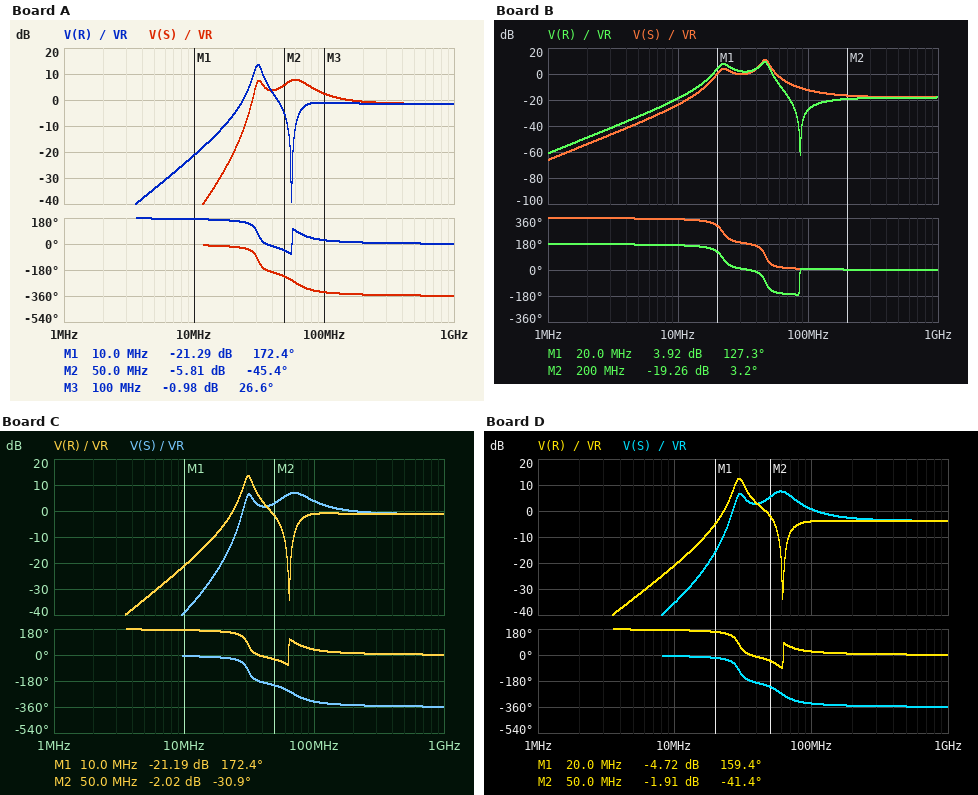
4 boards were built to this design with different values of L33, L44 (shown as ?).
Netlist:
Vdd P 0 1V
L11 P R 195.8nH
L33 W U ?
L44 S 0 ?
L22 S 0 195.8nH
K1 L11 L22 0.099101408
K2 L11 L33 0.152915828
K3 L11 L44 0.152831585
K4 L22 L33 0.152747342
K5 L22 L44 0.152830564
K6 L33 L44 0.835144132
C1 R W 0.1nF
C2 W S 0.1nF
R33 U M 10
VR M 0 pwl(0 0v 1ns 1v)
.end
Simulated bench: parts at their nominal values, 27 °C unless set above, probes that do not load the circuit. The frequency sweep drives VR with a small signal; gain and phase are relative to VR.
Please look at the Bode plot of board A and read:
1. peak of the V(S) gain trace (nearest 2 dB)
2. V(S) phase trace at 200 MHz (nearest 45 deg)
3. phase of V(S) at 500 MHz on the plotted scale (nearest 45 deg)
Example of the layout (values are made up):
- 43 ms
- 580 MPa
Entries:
- 8 dB
- -360 deg
- -360 deg
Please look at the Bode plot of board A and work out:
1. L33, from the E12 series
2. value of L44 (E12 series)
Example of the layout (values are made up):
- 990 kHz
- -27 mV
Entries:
- 82 nH
- 330 nH
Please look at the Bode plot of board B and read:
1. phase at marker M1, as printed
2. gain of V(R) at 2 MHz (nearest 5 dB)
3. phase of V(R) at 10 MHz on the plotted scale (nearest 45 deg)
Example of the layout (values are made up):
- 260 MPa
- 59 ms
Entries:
- 127.3 deg
- -50 dB
- 180 deg
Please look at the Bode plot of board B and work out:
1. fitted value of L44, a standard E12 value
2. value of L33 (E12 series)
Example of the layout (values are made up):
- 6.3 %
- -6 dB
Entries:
- 560 nH
- 470 nH
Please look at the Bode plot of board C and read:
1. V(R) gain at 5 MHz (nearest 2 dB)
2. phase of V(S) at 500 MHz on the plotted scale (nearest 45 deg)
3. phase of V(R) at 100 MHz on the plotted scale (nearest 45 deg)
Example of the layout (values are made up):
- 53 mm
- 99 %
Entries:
- -34 dB
- -360 deg
- 45 deg
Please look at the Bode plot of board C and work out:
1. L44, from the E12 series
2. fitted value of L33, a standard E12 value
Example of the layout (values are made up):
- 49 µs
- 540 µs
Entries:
- 220 nH
- 68 nH
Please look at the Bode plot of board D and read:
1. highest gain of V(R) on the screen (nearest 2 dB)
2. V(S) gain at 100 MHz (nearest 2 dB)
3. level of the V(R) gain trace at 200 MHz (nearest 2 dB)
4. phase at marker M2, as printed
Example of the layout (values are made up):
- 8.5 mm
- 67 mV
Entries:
- 12 dB
- 0 dB
- -4 dB
- -41.4 deg
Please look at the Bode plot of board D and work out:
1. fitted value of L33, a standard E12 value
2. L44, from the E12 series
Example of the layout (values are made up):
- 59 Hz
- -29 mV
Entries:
- 120 nH
- 330 nH
